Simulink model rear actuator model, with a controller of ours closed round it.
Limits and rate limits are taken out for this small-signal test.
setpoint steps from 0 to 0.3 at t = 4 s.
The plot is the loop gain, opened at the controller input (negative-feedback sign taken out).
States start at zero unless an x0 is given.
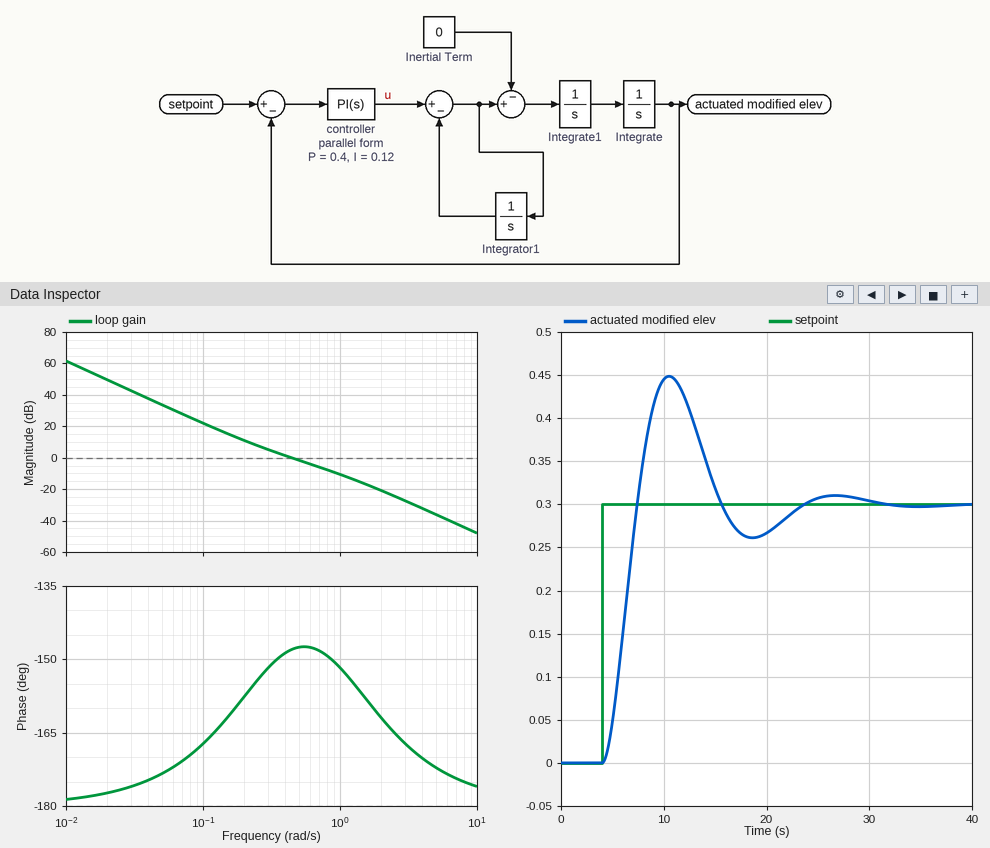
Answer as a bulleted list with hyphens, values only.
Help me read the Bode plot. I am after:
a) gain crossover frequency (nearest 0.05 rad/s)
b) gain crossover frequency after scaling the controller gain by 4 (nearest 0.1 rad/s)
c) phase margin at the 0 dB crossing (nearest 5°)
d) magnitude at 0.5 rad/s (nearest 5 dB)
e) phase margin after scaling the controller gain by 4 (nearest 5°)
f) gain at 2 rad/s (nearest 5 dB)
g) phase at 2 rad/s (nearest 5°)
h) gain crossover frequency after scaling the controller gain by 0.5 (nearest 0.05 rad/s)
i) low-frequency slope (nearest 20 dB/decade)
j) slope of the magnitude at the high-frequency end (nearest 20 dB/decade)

- 0.45 rad/s
- 1.1 rad/s
- 30°
- 0 dB
- 25°
- -20 dB
- -160°
- 0.30 rad/s
- -40 dB/decade
- -40 dB/decade
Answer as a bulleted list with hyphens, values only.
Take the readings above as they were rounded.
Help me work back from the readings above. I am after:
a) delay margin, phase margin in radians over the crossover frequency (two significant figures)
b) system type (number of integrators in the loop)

- 1.2 s
- 2
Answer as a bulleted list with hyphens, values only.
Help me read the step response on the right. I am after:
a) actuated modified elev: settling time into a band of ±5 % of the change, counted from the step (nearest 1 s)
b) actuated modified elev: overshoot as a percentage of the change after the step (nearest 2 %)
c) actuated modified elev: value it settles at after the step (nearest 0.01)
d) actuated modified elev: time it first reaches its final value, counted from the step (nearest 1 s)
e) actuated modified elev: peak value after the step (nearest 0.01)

- 18 s
- 50 %
- 0.30
- 3 s
- 0.45
